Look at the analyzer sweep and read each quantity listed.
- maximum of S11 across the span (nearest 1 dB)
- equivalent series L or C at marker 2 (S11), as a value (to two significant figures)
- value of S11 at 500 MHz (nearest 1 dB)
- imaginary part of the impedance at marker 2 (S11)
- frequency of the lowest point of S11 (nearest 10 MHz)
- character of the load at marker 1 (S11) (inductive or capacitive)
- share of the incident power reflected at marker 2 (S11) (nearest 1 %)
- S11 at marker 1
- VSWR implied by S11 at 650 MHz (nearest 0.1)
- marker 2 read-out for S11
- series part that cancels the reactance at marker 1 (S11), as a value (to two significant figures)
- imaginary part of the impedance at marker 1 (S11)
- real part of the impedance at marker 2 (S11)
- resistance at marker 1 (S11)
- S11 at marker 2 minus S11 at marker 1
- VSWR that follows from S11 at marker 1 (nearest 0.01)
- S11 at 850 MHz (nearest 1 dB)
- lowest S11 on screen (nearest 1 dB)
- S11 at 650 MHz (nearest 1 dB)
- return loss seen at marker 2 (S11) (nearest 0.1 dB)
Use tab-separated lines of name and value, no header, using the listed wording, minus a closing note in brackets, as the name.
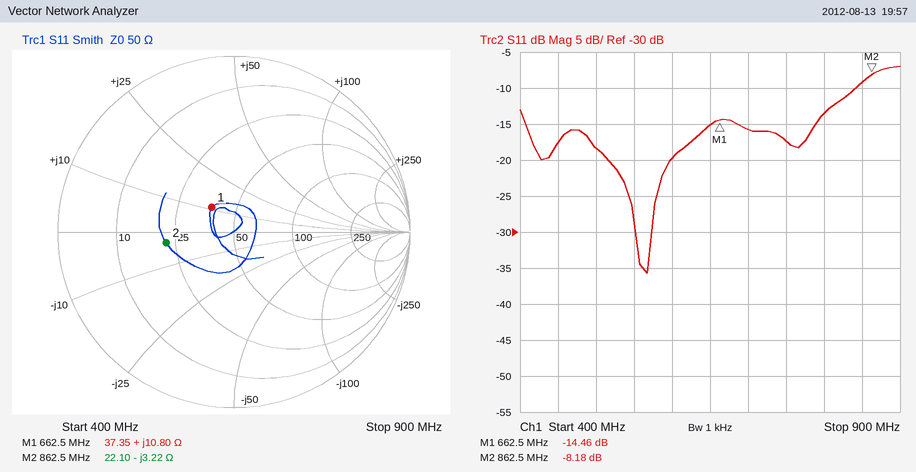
maximum of S11 across the span	-7 dB
equivalent series L or C at marker 2 (S11), as a value	57 pF
value of S11 at 500 MHz	-18 dB
imaginary part of the impedance at marker 2	-3.22 Ω
frequency of the lowest point of S11	570 MHz
character of the load at marker 1 (S11)	inductive
share of the incident power reflected at marker 2 (S11)	15 %
S11 at marker 1	-14.46 dB
VSWR implied by S11 at 650 MHz	1.4
marker 2 read-out for S11	-8.18 dB
series part that cancels the reactance at marker 1 (S11), as a value	22 pF
imaginary part of the impedance at marker 1	+10.80 Ω
real part of the impedance at marker 2	22.10 Ω
resistance at marker 1	37.35 Ω
S11 at marker 2 minus S11 at marker 1	6.28 dB
VSWR that follows from S11 at marker 1	1.47
S11 at 850 MHz	-9 dB
lowest S11 on screen	-36 dB
S11 at 650 MHz	-15 dB
return loss seen at marker 2 (S11)	8.2 dB
